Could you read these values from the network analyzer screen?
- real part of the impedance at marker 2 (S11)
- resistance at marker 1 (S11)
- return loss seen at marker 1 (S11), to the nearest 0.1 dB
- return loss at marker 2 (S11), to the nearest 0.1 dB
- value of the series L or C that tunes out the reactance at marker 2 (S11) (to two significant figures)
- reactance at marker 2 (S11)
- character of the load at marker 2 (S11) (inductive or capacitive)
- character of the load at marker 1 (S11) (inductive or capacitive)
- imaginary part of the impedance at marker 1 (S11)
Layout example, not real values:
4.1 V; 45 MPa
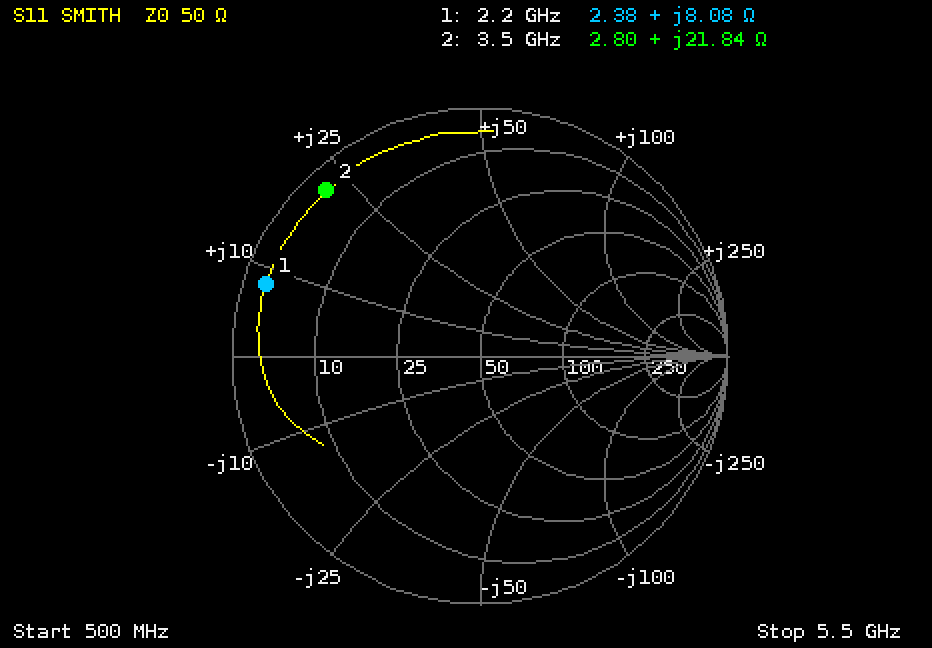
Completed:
2.80 Ω; 2.38 Ω; 0.8 dB; 0.8 dB; 2.1 pF; +21.84 Ω; inductive; inductive; +8.08 Ω
